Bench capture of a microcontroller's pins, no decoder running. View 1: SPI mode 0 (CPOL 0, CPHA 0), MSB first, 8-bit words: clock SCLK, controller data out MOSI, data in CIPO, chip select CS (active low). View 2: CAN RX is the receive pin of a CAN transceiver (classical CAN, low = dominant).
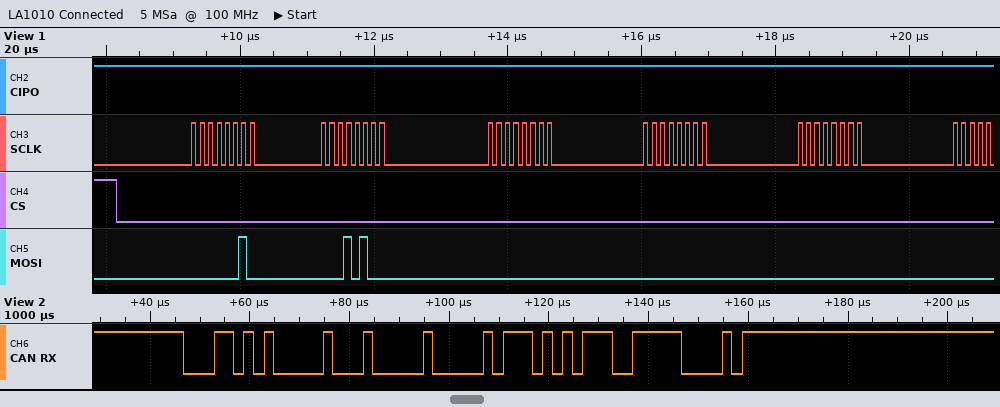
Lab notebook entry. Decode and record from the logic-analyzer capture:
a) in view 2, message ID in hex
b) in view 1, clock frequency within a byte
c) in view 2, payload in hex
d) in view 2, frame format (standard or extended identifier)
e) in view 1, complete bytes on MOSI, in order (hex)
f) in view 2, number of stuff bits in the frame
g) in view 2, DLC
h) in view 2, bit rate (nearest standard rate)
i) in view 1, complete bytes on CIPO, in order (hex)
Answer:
0x1A8
8 MHz
00 3A
standard
0x02 0x14 0x00 0x00 0x00
4
2
500 kbit/s
0xFF 0xFF 0xFF 0xFF 0xFF
